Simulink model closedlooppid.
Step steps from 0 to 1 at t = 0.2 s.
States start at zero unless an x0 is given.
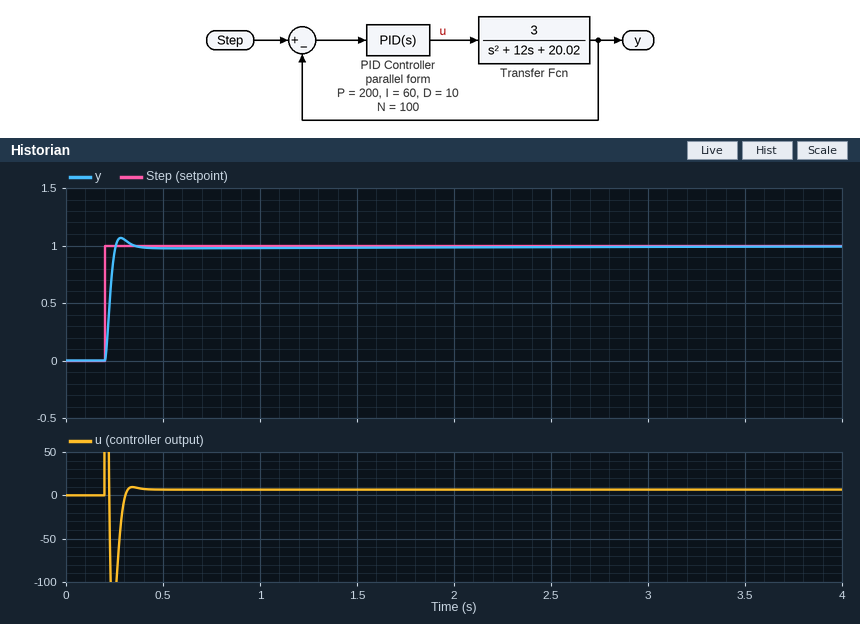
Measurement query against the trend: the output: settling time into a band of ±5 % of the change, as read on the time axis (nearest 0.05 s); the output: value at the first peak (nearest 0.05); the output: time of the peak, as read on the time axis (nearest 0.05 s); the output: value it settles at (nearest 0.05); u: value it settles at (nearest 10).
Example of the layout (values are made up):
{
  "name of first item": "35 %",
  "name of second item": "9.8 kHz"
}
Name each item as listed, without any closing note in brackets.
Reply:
{
  "the output: settling time into a band of ±5 % of the change, as read on the time axis": "0.30 s",
  "the output: value at the first peak": "1.05",
  "the output: time of the peak, as read on the time axis": "0.30 s",
  "the output: value it settles at": "1.00",
  "u: value it settles at": "10"
}
